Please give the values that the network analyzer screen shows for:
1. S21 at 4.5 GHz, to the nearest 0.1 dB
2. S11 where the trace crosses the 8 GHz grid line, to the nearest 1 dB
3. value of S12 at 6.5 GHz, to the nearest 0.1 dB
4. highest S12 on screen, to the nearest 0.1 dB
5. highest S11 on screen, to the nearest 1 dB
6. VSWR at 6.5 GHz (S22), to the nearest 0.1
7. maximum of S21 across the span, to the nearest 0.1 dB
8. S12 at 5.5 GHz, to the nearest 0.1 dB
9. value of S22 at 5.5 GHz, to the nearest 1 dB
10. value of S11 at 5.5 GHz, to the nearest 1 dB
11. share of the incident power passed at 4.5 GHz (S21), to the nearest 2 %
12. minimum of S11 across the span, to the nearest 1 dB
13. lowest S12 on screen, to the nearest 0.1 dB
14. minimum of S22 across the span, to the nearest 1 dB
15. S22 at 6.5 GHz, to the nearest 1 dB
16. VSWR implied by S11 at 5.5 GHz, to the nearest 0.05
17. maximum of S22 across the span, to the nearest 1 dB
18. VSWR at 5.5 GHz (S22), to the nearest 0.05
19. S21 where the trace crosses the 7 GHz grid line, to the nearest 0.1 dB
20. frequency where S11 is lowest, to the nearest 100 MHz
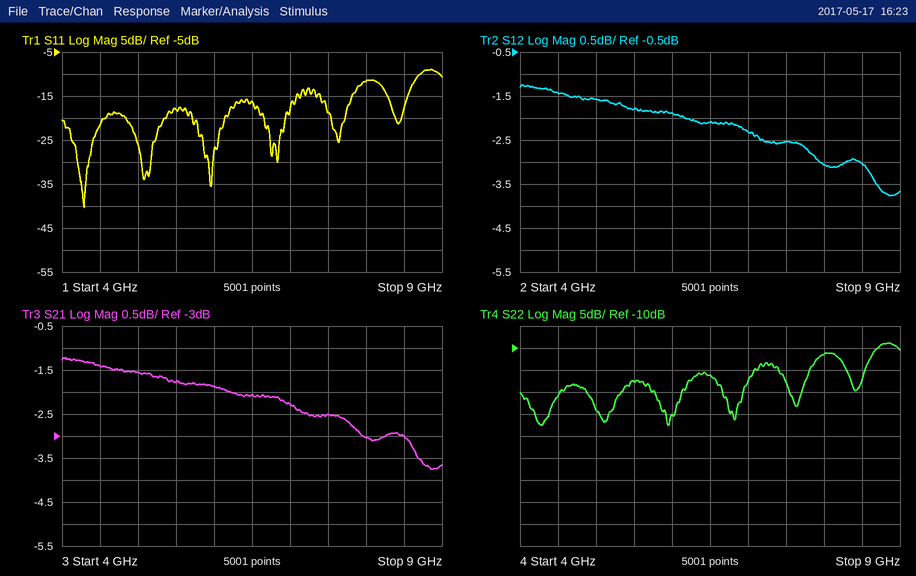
-1.4 dB
-12 dB
-2.1 dB
-1.2 dB
-9 dB
1.4
-1.2 dB
-1.8 dB
-18 dB
-18 dB
72 %
-40 dB
-3.8 dB
-28 dB
-16 dB
1.30
-9 dB
1.30
-2.3 dB
4.3 GHz
